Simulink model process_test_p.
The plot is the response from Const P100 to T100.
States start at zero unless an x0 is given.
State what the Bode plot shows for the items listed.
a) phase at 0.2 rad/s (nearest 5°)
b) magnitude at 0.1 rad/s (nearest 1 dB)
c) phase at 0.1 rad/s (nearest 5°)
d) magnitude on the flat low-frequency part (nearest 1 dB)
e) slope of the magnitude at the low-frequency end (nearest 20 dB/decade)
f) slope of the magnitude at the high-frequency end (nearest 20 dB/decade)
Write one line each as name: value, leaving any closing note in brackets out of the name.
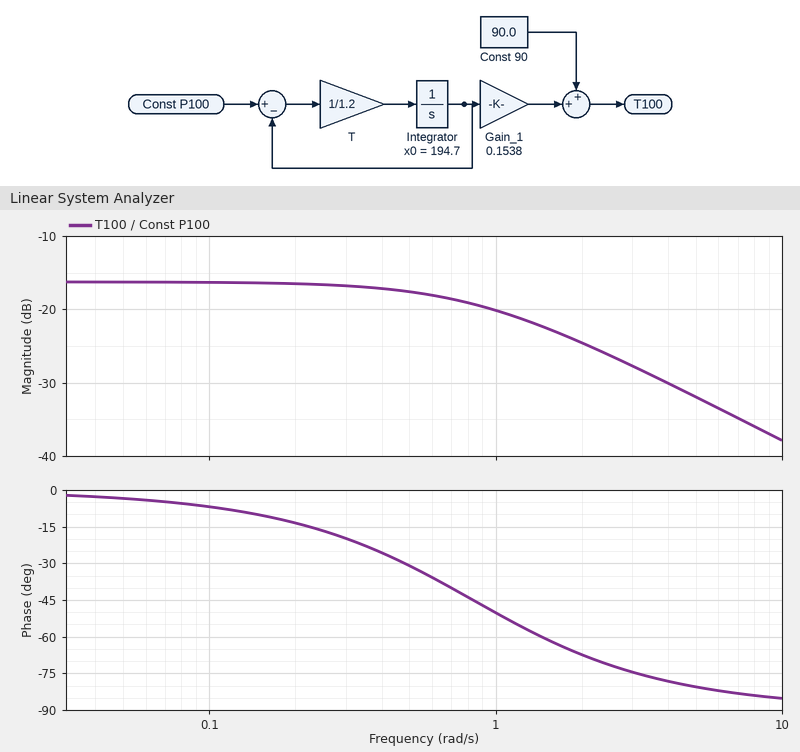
phase at 0.2 rad/s: -15°
magnitude at 0.1 rad/s: -16 dB
phase at 0.1 rad/s: -5°
magnitude on the flat low-frequency part: -16 dB
slope of the magnitude at the low-frequency end: 0 dB/decade
slope of the magnitude at the high-frequency end: -20 dB/decade
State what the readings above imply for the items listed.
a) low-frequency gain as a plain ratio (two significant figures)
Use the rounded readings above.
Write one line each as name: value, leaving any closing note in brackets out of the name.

low-frequency gain as a plain ratio: 0.16
